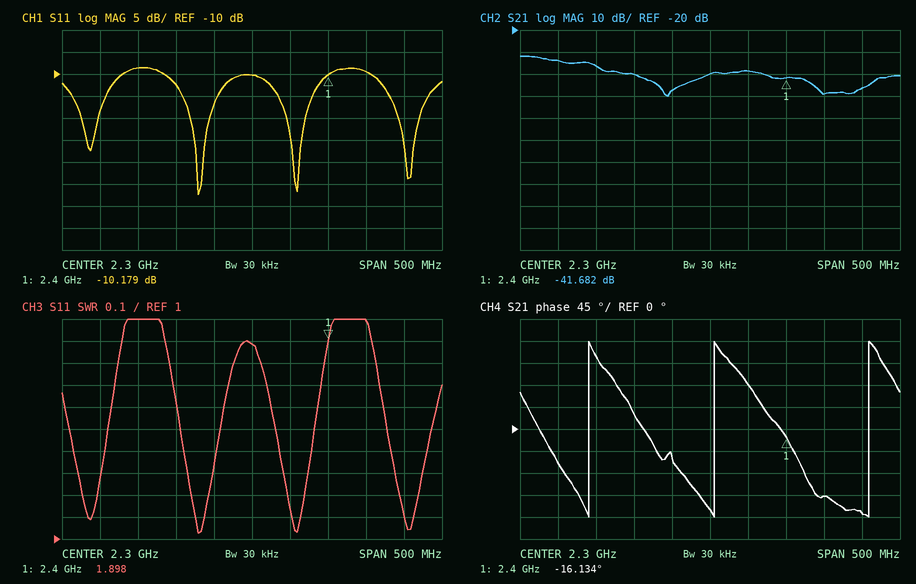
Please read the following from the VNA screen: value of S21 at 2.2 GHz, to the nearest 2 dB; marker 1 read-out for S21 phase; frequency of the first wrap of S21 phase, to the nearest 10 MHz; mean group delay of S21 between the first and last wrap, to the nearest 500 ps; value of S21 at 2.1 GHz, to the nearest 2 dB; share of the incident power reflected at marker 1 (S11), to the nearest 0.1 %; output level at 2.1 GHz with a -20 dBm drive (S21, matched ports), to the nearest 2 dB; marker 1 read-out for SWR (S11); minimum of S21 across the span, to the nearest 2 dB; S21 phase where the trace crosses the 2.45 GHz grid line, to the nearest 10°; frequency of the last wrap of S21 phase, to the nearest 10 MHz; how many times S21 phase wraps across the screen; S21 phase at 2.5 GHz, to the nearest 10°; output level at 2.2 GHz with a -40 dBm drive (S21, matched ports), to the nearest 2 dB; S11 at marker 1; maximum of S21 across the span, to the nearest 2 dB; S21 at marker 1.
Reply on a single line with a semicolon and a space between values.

-40 dB; -16.134°; 2.14 GHz; 5.5 ns; -34 dB; 9.6 %; -54 dBm; 1.898; -50 dB; -140°; 2.51 GHz; 3; -170°; -80 dBm; -10.179 dB; -32 dB; -41.682 dB
